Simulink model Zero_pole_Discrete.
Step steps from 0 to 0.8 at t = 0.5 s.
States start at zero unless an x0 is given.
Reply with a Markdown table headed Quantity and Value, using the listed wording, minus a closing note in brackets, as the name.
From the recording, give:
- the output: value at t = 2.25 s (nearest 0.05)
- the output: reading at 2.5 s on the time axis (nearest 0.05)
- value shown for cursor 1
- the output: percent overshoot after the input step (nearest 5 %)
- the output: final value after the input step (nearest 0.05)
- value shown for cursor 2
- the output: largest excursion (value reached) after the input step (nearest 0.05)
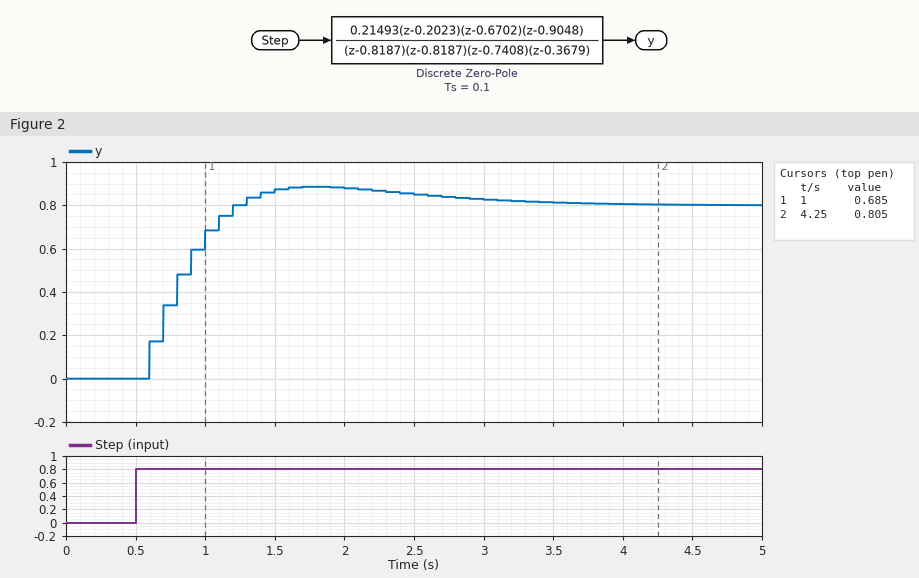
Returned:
| Quantity | Value |
|---|---|
| the output: value at t = 2.25 s | 0.85 |
| the output: reading at 2.5 s on the time axis | 0.85 |
| value shown for cursor 1 | 0.685 |
| the output: percent overshoot after the input step | 10 % |
| the output: final value after the input step | 0.80 |
| value shown for cursor 2 | 0.805 |
| the output: largest excursion (value reached) after the input step | 0.90 |
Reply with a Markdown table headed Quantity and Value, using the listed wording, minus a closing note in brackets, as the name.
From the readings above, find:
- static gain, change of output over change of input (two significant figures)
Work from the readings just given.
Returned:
| Quantity | Value |
|---|---|
| static gain, change of output over change of input | 1.0 |
